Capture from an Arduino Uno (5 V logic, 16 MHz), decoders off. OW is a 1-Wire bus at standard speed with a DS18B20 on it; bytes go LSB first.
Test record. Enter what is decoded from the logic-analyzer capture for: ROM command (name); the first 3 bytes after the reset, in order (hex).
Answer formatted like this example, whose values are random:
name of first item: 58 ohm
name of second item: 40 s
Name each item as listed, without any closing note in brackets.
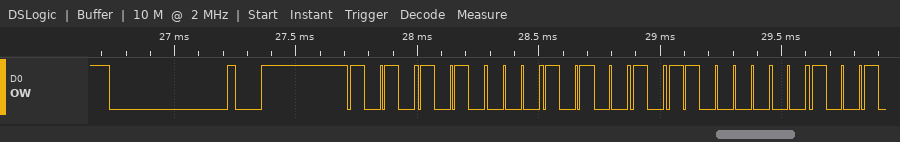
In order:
ROM command: Match ROM
the first 3 bytes after the reset, in order: 55 28 0D
